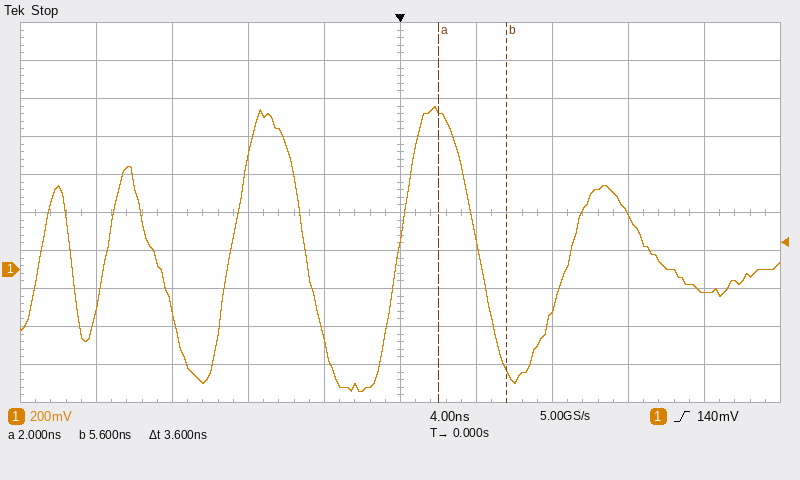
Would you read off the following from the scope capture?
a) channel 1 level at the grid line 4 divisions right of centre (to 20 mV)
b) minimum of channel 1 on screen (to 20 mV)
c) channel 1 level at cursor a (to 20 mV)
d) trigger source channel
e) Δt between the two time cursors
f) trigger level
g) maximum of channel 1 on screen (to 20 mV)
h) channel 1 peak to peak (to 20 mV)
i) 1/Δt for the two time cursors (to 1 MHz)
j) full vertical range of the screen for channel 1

-120 mV
-640 mV
840 mV
channel 1
3.6 ns
140 mV
860 mV
1.50 V
278 MHz
2 V
